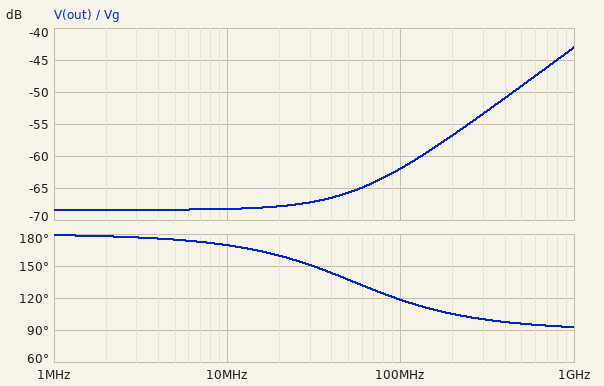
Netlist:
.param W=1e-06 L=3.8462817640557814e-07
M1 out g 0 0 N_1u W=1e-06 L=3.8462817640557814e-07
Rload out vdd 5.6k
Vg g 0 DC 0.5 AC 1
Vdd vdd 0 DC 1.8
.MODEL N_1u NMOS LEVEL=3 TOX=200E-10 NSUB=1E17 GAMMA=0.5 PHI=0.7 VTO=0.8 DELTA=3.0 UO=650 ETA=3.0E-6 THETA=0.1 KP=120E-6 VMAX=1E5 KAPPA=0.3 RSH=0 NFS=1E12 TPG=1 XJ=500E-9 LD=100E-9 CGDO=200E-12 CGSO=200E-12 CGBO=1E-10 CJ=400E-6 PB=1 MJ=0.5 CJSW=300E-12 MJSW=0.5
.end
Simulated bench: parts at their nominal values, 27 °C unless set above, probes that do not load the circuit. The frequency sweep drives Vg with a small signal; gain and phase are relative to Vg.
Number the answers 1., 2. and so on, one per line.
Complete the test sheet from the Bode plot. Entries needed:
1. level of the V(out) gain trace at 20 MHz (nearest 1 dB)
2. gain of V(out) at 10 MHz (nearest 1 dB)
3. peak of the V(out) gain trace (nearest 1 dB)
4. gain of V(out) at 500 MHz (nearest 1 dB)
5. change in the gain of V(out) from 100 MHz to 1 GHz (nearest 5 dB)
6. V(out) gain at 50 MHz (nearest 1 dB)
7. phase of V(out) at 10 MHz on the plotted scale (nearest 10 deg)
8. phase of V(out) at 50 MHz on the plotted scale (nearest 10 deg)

1. -68 dB
2. -68 dB
3. -43 dB
4. -49 dB
5. 20 dB
6. -66 dB
7. 170 deg
8. 140 deg
